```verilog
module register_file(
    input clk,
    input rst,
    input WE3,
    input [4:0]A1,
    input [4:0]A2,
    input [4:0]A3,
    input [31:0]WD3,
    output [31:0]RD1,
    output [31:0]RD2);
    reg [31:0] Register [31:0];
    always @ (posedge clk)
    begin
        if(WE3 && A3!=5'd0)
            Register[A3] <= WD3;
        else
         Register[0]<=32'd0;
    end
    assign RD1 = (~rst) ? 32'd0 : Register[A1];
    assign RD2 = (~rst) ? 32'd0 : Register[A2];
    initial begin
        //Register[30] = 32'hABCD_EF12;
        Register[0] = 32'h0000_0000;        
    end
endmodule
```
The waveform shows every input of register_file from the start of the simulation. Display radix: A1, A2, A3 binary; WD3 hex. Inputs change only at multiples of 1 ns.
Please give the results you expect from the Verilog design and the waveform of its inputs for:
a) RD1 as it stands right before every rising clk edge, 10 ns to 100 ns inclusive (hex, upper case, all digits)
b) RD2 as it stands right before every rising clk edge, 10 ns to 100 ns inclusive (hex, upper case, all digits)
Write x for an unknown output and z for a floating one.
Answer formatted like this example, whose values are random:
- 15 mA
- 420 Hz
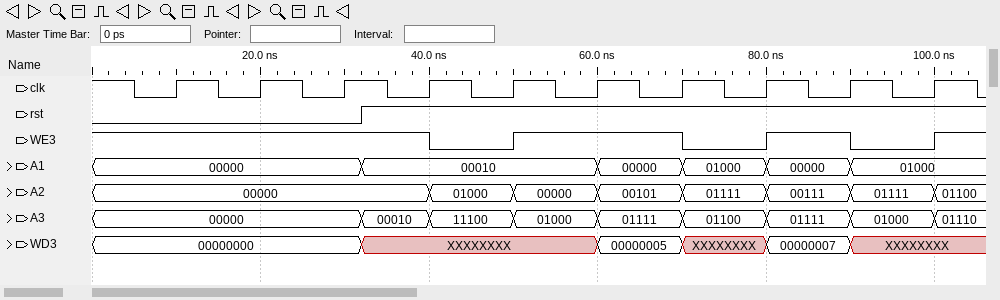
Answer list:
- 00000000, 00000000, 00000000, x, x, x, 00000000, x, 00000000, x
- 00000000, 00000000, 00000000, 00000000, x, 00000000, x, 00000005, x, 00000007
